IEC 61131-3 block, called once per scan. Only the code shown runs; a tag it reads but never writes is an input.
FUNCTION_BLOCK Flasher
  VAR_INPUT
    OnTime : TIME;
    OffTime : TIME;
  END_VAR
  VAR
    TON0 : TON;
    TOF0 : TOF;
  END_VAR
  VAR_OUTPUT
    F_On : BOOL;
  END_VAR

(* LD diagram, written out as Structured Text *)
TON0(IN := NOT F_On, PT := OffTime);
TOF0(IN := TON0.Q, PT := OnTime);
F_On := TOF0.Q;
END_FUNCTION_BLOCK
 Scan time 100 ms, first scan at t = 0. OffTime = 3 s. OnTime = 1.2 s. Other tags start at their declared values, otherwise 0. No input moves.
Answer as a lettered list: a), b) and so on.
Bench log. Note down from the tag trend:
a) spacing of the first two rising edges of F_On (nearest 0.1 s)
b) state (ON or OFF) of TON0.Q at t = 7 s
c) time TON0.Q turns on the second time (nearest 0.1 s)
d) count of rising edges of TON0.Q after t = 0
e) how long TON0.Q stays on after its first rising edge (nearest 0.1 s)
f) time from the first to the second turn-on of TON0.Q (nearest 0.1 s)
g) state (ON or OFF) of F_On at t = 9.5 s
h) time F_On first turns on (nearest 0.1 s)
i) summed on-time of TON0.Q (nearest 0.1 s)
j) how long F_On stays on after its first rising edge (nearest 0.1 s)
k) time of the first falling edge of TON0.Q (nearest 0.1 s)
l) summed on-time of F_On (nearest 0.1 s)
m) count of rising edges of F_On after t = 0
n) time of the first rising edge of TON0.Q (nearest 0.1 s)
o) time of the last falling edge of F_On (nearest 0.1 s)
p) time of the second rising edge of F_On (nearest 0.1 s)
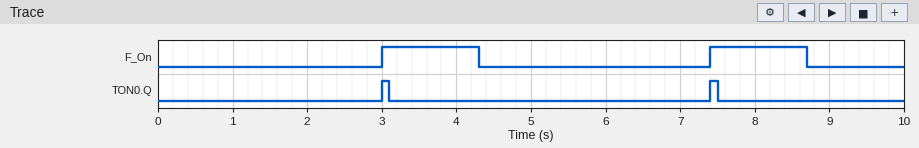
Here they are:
a) 4.4 s
b) OFF
c) 7.4 s
d) 2
e) 0.1 s
f) 4.4 s
g) OFF
h) 3.0 s
i) 0.2 s
j) 1.3 s
k) 3.1 s
l) 2.6 s
m) 2
n) 3.0 s
o) 8.7 s
p) 7.4 s
